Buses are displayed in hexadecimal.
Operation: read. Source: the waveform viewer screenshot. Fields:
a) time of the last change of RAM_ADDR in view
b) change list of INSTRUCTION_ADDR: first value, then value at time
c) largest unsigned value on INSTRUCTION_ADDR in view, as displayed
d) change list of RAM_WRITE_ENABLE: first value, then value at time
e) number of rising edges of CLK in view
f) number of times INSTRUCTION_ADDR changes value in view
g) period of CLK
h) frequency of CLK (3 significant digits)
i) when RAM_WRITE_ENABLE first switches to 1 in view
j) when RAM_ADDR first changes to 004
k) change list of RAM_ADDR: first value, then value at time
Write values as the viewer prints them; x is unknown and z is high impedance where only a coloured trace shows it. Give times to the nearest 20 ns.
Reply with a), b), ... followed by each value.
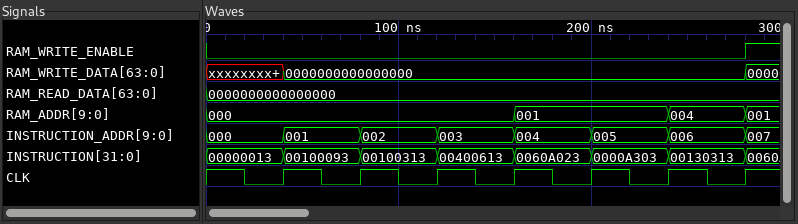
a) 280 ns
b) 000, 001 at 40 ns, 002 at 80 ns, 003 at 120 ns, 004 at 160 ns, 005 at 200 ns, 006 at 240 ns, 007 at 280 ns
c) 007
d) 0, 1 at 280 ns
e) 7
f) 7
g) 40 ns
h) 25.0 MHz
i) 280 ns
j) 240 ns
k) 000, 001 at 160 ns, 004 at 240 ns, 001 at 280 ns
